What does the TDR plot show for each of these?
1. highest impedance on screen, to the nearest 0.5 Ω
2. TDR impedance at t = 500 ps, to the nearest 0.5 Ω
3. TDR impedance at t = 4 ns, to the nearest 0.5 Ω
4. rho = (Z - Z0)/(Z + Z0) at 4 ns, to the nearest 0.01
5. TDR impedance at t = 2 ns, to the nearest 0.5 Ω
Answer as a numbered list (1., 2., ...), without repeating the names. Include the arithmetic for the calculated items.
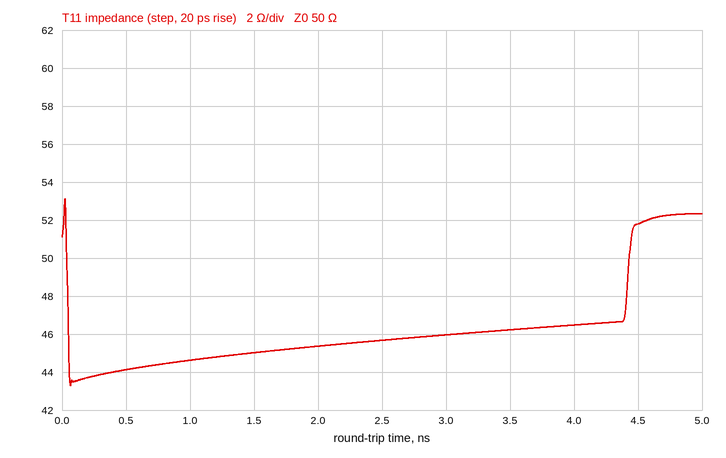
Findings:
1. 53.0 Ω
2. 44.0 Ω
3. 46.5 Ω
4. (46.5 − 50)/(46.5 + 50) ≈ -0.04
5. 45.5 Ω
